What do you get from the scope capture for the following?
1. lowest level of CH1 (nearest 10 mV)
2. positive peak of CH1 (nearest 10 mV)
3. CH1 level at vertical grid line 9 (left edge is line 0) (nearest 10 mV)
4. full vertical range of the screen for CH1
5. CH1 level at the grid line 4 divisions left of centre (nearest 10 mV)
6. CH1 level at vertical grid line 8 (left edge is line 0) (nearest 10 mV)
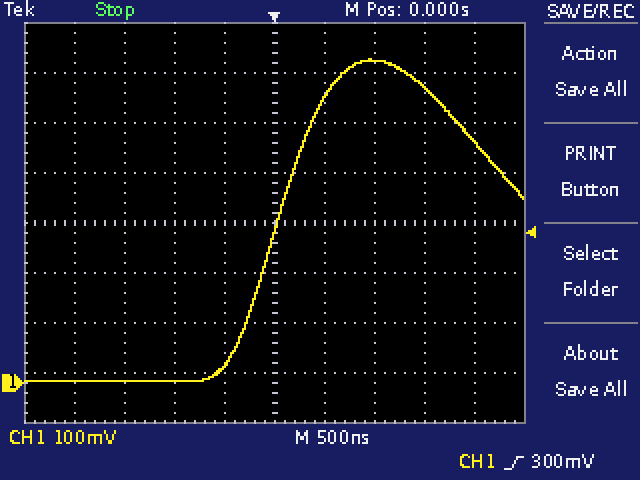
0 mV
650 mV
480 mV
800 mV
0 mV
590 mV
